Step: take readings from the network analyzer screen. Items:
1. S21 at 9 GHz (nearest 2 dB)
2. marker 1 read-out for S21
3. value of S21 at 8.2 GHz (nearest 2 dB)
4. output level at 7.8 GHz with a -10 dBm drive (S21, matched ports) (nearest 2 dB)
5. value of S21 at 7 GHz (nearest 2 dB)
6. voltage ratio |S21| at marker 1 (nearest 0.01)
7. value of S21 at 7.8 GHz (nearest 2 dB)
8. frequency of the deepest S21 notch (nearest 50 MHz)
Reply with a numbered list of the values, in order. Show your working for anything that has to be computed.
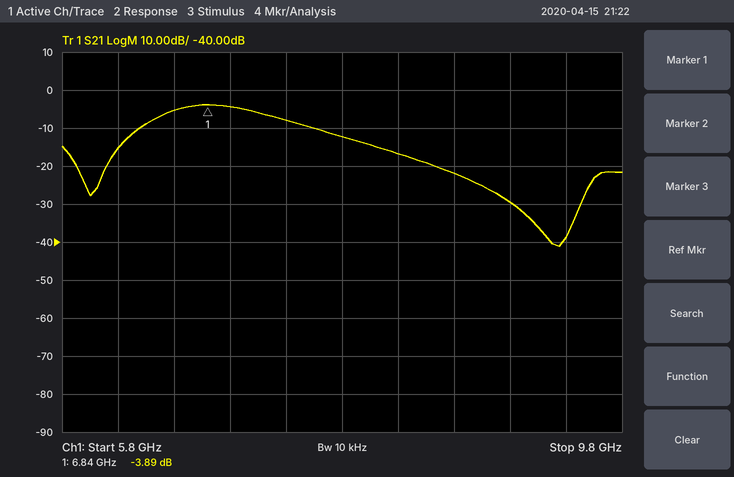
1. -30 dB
2. -3.89 dB
3. -16 dB
4. -10 dBm + (-12 dB) = -22 dBm
5. -4 dB
6. 10^(-3.89/20) ≈ 0.64
7. -12 dB
8. 9.35 GHz
